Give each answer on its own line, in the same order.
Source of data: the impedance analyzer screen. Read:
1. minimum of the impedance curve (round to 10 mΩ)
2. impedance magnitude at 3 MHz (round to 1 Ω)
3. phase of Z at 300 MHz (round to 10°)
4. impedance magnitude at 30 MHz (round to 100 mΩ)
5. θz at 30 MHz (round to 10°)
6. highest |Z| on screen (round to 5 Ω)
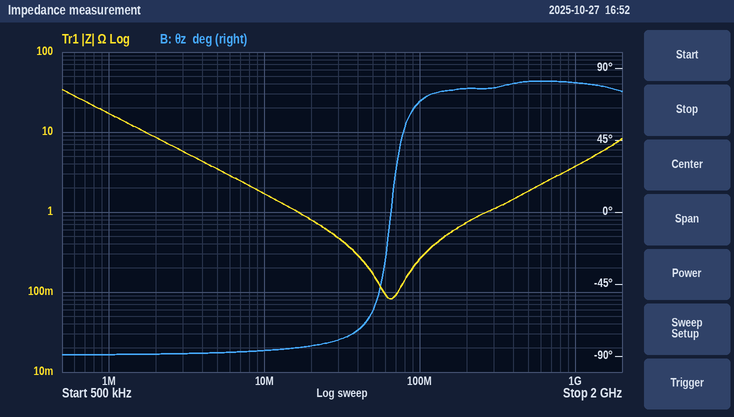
80 mΩ
6 Ω
80°
500 mΩ
-80°
35 Ω
